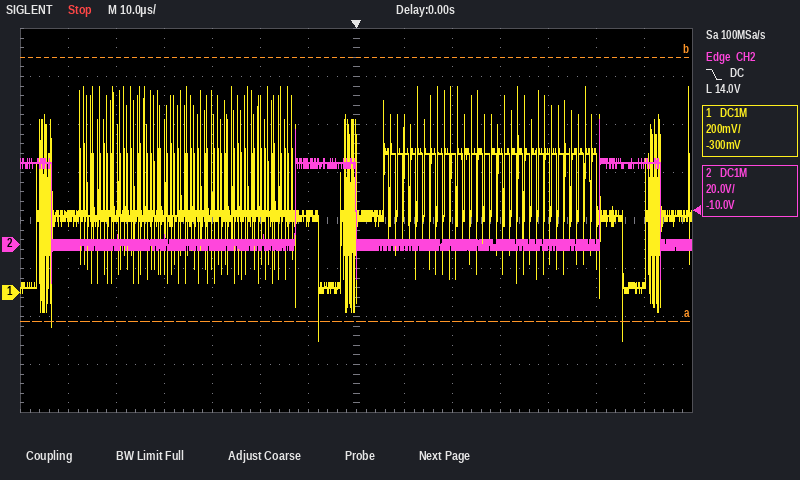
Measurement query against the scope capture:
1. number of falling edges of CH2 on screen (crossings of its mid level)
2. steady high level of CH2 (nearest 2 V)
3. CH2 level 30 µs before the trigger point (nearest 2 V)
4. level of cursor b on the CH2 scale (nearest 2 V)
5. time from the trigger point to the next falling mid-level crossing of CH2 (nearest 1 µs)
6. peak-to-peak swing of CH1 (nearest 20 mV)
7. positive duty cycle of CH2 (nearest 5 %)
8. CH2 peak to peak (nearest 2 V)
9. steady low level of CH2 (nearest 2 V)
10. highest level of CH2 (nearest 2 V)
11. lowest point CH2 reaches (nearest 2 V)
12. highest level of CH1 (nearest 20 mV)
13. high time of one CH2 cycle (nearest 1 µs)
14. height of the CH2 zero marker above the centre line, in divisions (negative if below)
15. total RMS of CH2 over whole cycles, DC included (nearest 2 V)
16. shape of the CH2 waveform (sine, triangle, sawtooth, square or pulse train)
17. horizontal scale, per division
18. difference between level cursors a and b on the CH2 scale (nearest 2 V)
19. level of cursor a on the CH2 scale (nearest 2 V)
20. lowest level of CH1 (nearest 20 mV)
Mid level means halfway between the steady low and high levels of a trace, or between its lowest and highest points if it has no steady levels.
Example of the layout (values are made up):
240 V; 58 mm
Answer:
3; 34 V; 0 V; 78 V; 63 µs; 1.06 V; 20 %; 68 V; 0 V; 52 V; -16 V; 860 mV; 13 µs; -0.5 div; 16 V; pulse train; 10 µs; 110 V; -32 V; -200 mV
